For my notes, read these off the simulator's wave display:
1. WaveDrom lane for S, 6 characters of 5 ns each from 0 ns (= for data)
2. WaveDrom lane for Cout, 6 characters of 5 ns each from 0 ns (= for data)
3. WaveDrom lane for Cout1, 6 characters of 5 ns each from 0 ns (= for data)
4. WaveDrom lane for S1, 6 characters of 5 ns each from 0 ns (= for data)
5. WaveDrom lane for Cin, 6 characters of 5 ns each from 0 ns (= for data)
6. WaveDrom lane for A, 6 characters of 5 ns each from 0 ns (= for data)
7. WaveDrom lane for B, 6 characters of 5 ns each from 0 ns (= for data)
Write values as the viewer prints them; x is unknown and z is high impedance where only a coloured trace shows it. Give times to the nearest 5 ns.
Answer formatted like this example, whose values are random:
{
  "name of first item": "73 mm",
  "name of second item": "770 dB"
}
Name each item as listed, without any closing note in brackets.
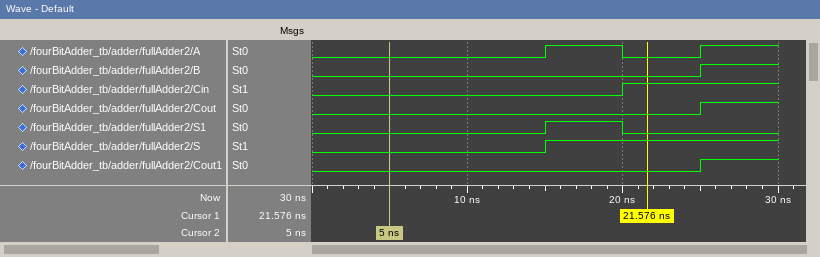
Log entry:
{
  "WaveDrom lane for S, 6 characters of 5 ns each from 0 ns": "{name: 'S', wave: '0..1..'}",
  "WaveDrom lane for Cout, 6 characters of 5 ns each from 0 ns": "{name: 'Cout', wave: '0....1'}",
  "WaveDrom lane for Cout1, 6 characters of 5 ns each from 0 ns": "{name: 'Cout1', wave: '0....1'}",
  "WaveDrom lane for S1, 6 characters of 5 ns each from 0 ns": "{name: 'S1', wave: '0..10.'}",
  "WaveDrom lane for Cin, 6 characters of 5 ns each from 0 ns": "{name: 'Cin', wave: '0...1.'}",
  "WaveDrom lane for A, 6 characters of 5 ns each from 0 ns": "{name: 'A', wave: '0..101'}",
  "WaveDrom lane for B, 6 characters of 5 ns each from 0 ns": "{name: 'B', wave: '0....1'}"
}
